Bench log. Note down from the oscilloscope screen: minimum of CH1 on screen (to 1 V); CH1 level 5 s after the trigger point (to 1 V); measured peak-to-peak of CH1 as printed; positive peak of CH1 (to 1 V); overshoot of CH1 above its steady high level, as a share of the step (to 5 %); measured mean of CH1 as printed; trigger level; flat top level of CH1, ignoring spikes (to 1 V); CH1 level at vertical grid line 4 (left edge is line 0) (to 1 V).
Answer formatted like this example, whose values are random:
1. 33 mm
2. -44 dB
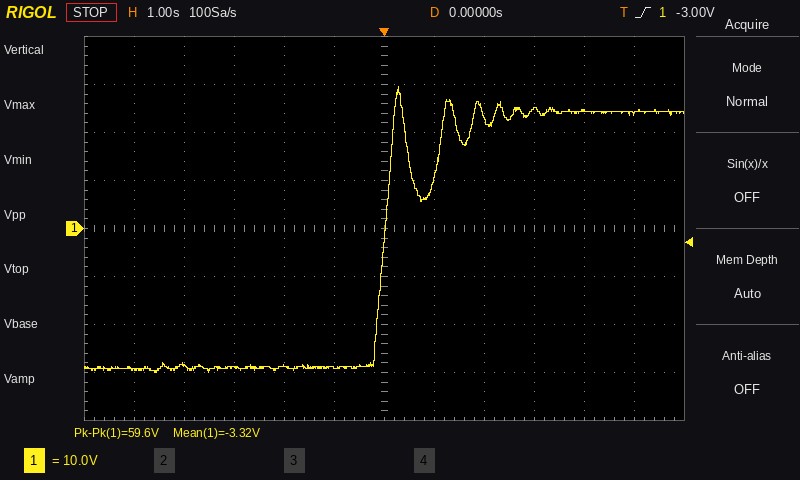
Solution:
1. -30 V
2. 24 V
3. 59.6 V
4. 30 V
5. 10 %
6. -3.32 V
7. -3.00 V
8. 24 V
9. -29 V
